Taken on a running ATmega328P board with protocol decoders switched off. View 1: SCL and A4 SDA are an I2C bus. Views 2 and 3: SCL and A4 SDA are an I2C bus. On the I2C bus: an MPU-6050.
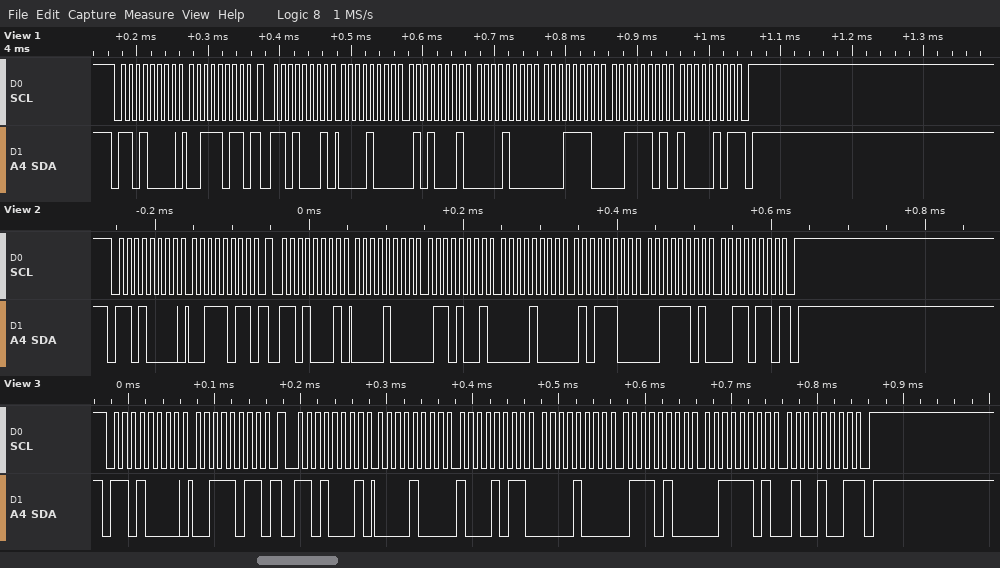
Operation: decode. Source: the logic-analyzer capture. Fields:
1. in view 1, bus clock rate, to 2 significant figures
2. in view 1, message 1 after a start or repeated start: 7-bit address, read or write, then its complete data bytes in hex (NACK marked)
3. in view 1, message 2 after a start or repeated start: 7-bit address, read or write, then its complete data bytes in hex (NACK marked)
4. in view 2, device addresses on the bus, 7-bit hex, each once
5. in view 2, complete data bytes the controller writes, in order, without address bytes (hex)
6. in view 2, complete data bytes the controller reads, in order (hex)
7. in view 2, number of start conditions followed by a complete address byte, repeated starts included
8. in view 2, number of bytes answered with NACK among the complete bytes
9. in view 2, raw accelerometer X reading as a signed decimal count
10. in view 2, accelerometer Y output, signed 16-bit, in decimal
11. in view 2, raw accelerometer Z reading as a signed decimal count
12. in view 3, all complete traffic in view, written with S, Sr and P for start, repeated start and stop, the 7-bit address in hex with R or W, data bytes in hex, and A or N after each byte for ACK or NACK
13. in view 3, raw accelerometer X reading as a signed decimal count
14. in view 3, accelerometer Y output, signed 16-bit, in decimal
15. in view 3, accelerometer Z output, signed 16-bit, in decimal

100 kHz
0x68 write: 3B
0x68 read: 08 51 08 1E 3D 85 NACK
0x68
3B
08 69 08 5C 3D 36
2
1
2153
2140
15670
S 68W A 3B A Sr 68R A 08 A 8B A 08 A 74 A 3D A 49 N P
2187
2164
15689
